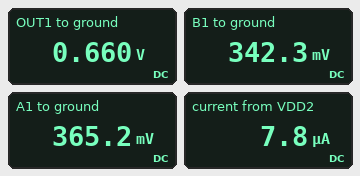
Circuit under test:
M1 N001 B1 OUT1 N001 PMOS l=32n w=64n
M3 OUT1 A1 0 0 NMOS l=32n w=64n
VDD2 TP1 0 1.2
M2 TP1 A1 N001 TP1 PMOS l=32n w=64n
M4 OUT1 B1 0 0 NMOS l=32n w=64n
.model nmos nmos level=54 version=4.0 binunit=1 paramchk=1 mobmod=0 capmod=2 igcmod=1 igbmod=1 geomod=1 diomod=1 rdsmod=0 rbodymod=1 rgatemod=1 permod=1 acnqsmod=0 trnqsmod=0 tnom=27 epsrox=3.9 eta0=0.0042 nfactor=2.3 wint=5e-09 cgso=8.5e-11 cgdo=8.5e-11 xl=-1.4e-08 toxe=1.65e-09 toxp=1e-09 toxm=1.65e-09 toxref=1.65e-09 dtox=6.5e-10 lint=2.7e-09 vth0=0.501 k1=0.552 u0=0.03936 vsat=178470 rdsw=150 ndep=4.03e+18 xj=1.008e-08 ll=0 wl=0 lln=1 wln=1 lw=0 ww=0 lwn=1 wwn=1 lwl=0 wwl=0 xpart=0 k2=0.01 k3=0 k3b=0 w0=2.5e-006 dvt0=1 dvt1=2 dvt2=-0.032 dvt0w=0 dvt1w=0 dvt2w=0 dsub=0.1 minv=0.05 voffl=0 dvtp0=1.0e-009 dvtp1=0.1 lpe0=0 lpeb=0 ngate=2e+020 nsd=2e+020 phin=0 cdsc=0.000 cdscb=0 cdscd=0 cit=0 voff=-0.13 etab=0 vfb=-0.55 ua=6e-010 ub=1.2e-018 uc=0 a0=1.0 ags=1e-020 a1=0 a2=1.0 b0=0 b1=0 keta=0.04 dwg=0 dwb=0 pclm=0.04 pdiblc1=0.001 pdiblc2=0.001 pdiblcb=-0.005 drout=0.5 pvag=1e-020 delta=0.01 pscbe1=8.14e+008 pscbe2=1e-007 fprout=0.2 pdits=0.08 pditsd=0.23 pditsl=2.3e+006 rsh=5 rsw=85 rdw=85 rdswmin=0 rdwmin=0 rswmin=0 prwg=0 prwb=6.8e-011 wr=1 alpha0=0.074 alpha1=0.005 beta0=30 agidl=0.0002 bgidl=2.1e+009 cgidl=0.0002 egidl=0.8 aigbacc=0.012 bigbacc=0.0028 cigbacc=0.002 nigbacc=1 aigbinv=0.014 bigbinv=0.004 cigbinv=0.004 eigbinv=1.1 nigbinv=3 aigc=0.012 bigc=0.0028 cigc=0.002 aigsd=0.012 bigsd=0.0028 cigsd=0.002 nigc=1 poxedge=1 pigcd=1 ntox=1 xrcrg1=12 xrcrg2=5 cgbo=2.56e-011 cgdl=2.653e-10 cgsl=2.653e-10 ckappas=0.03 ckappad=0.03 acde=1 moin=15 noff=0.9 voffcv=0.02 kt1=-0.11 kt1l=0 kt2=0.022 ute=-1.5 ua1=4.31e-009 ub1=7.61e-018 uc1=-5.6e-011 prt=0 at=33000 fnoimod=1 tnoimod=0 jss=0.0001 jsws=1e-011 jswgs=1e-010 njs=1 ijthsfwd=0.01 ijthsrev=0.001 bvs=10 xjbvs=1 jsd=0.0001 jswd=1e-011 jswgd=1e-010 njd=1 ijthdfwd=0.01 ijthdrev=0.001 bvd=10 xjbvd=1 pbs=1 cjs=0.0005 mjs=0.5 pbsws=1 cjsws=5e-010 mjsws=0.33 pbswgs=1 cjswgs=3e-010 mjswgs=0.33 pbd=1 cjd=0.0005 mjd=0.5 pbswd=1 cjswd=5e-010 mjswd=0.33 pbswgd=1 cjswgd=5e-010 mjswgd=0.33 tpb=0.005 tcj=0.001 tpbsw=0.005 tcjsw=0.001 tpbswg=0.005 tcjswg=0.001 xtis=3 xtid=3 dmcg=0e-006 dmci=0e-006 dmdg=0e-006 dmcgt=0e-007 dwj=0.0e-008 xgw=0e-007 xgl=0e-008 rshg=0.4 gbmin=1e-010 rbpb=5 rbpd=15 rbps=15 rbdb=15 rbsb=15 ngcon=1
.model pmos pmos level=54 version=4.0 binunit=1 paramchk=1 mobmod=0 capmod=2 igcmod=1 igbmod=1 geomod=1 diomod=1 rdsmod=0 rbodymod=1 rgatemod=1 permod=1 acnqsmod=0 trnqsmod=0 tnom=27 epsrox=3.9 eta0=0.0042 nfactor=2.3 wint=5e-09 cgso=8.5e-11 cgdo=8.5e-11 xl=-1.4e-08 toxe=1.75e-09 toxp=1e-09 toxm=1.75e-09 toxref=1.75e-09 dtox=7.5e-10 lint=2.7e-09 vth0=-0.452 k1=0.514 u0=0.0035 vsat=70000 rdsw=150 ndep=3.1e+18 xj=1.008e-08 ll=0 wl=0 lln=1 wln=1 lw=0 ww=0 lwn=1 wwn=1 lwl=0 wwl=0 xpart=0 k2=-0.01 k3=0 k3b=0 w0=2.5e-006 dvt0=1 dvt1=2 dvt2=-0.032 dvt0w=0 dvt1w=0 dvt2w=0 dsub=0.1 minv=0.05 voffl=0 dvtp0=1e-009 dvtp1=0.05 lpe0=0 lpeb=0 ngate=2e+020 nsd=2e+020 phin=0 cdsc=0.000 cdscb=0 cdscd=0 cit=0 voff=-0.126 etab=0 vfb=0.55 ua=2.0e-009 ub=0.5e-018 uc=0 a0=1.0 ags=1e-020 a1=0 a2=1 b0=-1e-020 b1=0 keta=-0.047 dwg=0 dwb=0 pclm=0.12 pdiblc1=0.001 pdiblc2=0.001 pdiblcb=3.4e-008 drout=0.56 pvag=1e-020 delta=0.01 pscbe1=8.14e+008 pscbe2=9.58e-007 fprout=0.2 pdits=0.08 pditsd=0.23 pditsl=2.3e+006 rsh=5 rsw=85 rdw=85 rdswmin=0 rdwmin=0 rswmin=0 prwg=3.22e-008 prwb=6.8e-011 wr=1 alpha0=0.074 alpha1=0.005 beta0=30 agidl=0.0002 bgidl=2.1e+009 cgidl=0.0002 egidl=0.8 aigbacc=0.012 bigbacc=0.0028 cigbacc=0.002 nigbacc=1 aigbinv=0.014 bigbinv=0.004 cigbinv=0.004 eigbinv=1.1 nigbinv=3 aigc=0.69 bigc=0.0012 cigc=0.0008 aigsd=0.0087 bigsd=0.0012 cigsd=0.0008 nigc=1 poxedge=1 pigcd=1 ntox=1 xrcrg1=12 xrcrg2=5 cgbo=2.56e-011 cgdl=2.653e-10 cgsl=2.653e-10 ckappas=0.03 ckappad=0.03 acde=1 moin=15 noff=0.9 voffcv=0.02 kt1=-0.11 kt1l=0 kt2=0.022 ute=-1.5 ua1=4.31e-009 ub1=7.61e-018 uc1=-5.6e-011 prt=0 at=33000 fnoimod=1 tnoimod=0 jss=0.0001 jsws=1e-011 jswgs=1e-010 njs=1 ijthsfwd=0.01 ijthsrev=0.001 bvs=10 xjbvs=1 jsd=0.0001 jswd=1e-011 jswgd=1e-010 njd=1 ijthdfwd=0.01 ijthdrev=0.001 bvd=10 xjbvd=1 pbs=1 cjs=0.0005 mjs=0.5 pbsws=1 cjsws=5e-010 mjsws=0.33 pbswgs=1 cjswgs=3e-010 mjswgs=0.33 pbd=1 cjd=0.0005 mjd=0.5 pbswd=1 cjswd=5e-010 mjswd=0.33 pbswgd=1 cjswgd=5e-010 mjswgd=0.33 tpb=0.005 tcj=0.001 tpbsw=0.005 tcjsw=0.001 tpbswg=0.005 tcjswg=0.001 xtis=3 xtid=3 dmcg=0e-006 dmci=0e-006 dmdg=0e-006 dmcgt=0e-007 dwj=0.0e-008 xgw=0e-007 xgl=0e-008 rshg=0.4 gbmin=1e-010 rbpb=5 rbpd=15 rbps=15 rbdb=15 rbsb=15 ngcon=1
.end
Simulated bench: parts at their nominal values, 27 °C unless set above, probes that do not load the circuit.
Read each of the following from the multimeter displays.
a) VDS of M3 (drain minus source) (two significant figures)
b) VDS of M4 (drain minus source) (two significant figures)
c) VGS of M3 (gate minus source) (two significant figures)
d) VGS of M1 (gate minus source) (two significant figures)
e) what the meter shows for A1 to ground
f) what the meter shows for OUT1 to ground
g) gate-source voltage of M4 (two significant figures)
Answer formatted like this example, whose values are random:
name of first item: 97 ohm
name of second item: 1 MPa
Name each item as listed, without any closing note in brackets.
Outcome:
VDS of M3 (drain minus source): 660 mV
VDS of M4 (drain minus source): 660 mV
VGS of M3 (gate minus source): 370 mV
VGS of M1 (gate minus source): -320 mV
what the meter shows for A1 to ground: 365.2 mV
what the meter shows for OUT1 to ground: 0.660 V
gate-source voltage of M4: 340 mV
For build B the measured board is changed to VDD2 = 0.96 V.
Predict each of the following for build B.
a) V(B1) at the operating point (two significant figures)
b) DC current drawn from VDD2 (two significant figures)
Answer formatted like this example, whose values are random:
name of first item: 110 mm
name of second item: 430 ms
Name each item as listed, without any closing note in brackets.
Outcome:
V(B1) at the operating point: 300 mV
DC current drawn from VDD2: 2.8 µA
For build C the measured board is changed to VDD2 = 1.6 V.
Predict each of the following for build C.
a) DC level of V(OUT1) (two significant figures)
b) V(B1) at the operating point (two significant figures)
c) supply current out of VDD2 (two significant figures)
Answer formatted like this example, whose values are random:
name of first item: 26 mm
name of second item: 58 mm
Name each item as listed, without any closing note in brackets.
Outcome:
DC level of V(OUT1): 700 mV
V(B1) at the operating point: 380 mV
supply current out of VDD2: 20 µA
